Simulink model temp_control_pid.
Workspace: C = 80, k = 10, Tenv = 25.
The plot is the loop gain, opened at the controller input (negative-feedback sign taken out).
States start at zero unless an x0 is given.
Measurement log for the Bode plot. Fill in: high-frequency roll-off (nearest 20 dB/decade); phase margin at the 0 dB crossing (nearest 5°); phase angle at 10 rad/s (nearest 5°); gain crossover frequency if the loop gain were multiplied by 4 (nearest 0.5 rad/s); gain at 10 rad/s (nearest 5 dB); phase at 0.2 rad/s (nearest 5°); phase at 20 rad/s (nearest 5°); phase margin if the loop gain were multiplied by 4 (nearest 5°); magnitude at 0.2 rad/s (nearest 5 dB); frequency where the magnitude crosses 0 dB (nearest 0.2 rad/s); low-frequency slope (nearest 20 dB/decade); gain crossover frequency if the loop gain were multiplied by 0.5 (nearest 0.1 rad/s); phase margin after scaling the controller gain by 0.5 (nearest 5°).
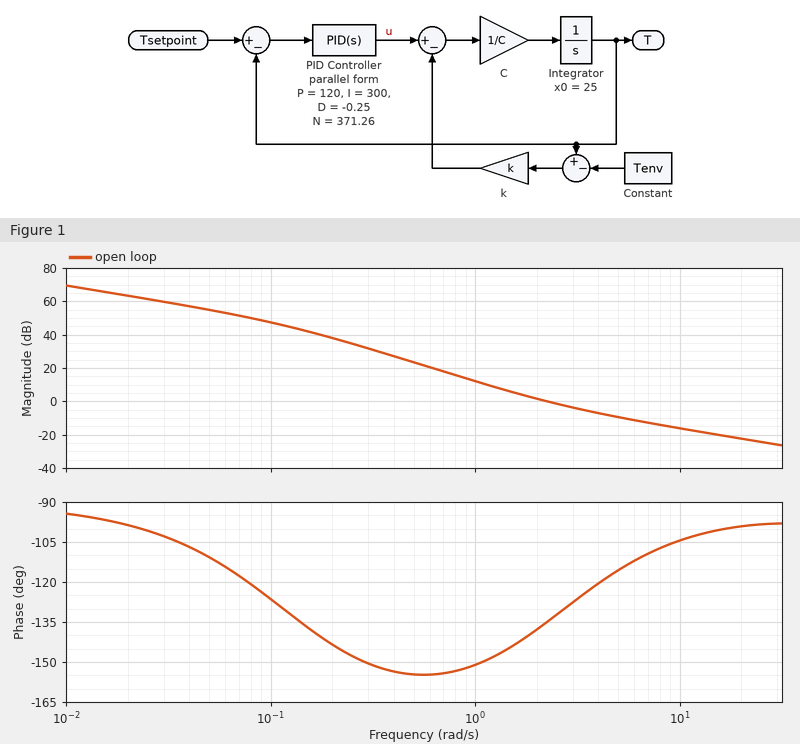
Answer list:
-20 dB/decade
45°
-105°
6.5 rad/s
-15 dB
-145°
-100°
70°
40 dB
2.2 rad/s
-20 dB/decade
1.5 rad/s
35°
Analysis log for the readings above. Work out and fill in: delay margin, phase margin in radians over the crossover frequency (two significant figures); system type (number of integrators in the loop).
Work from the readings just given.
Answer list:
0.36 s
1
